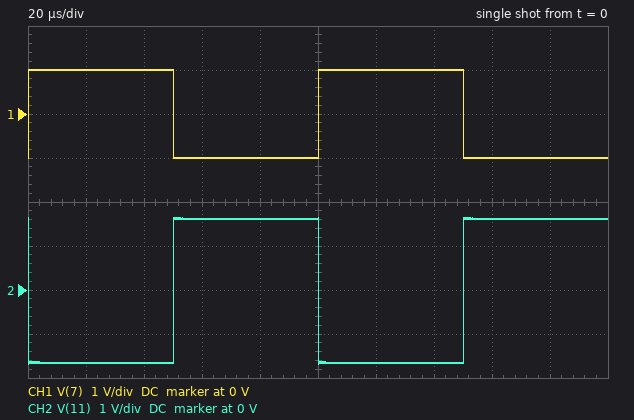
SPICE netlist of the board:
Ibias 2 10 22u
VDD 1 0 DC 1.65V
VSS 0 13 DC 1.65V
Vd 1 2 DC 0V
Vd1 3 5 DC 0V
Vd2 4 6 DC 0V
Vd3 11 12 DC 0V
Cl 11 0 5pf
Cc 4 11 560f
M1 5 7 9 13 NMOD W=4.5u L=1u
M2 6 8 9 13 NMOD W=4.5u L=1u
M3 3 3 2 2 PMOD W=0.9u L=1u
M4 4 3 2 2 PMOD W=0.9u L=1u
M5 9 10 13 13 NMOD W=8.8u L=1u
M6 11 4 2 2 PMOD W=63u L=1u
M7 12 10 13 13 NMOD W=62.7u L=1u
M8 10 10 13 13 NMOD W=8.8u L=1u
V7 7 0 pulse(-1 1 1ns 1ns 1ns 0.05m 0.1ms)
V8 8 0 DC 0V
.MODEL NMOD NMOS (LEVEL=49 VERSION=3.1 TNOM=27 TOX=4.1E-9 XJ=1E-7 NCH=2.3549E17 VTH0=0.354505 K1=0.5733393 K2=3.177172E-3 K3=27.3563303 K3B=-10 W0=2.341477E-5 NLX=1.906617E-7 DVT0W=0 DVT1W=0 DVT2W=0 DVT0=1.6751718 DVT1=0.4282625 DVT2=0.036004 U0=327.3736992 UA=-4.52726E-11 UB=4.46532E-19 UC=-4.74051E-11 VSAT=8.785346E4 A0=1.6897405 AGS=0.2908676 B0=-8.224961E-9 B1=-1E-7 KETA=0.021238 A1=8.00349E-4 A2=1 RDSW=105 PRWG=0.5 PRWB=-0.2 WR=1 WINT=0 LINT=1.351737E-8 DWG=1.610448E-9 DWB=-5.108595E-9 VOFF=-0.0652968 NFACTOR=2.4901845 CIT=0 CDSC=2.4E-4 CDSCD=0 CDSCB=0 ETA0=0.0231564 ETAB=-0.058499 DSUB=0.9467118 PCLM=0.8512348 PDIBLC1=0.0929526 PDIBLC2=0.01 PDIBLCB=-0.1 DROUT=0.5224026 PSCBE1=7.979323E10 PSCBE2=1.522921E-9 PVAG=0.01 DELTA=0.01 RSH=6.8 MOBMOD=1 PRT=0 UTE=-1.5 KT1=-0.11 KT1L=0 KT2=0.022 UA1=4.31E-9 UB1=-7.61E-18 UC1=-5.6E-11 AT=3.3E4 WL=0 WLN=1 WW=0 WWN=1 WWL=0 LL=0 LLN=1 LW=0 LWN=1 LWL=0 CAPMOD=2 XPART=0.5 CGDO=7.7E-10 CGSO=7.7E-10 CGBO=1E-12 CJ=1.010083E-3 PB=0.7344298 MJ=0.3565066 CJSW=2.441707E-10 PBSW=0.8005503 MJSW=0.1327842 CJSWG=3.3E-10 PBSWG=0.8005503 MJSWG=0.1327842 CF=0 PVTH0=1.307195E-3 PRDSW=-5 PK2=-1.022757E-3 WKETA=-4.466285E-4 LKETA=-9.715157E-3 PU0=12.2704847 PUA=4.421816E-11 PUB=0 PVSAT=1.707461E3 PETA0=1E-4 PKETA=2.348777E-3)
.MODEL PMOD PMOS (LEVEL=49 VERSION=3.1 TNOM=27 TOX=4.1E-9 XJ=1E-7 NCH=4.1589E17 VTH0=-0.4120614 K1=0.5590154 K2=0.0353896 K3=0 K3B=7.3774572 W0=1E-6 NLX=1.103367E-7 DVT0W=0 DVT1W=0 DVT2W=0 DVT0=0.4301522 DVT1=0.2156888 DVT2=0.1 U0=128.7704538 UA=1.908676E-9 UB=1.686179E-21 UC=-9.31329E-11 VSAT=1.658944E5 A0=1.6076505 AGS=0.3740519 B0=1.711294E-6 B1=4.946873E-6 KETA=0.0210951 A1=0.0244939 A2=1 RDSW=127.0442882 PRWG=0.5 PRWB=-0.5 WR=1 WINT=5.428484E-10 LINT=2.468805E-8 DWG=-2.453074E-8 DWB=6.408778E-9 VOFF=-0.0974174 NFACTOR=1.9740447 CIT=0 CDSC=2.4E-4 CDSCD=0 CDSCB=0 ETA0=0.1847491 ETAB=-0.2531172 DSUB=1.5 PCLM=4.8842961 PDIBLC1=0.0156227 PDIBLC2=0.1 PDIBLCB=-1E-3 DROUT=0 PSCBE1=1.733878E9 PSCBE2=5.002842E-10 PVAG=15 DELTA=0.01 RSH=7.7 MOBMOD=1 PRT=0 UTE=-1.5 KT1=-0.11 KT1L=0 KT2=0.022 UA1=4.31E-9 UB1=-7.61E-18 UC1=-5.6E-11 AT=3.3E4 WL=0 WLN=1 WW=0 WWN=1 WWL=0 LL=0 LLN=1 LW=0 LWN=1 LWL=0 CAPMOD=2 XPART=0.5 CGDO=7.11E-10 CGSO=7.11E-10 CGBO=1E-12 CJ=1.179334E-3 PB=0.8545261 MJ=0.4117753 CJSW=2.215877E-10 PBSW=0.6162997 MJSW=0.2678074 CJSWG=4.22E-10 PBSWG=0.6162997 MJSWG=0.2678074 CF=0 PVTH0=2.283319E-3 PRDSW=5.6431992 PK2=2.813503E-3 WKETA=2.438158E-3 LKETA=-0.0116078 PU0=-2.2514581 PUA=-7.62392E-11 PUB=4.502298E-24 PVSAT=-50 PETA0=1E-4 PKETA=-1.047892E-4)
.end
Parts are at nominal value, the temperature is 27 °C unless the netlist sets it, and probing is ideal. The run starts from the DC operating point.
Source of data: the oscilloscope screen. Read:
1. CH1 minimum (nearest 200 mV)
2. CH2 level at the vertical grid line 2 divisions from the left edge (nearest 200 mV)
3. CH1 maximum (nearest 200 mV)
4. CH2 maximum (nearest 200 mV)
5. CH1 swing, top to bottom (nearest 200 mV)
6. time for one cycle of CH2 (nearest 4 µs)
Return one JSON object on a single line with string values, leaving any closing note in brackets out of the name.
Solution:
{"CH1 minimum": "-1.0 V", "CH2 level at the vertical grid line 2 divisions from the left edge": "-1.6 V", "CH1 maximum": "1.0 V", "CH2 maximum": "1.6 V", "CH1 swing, top to bottom": "2.0 V", "time for one cycle of CH2": "100 µs"}
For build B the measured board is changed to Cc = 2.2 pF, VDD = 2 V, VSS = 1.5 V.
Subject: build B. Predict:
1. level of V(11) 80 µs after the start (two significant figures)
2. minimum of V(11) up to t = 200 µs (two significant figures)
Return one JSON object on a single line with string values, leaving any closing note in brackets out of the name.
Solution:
{"level of V(11) 80 µs after the start": "2.0 V", "minimum of V(11) up to t = 200 µs": "-1.5 V"}
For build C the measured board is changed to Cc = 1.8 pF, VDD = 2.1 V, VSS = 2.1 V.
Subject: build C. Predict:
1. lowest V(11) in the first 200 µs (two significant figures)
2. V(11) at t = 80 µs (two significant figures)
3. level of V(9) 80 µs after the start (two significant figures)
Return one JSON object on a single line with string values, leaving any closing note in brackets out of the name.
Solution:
{"lowest V(11) in the first 200 µs": "-2.1 V", "V(11) at t = 80 µs": "2.1 V", "level of V(9) 80 µs after the start": "-1.7 V"}
